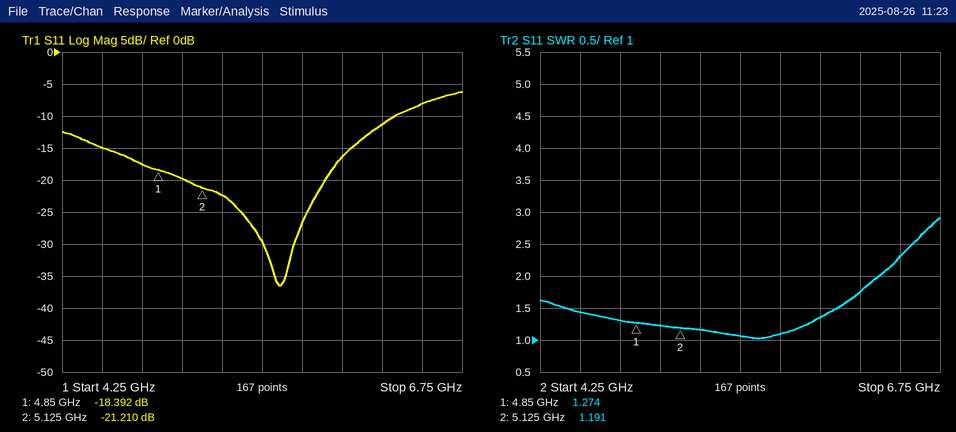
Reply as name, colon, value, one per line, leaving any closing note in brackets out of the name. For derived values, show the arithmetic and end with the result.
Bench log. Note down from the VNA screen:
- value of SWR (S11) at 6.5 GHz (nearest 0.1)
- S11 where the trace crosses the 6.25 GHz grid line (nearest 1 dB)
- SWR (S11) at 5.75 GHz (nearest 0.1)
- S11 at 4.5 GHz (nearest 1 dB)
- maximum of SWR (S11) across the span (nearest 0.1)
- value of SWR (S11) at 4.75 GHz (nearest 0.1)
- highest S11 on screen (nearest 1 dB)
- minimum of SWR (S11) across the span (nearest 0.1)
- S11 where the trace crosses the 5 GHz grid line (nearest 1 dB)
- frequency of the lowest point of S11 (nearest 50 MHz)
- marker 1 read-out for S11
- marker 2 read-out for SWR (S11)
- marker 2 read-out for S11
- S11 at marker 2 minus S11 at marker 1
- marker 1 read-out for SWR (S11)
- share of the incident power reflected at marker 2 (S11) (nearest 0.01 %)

value of SWR (S11) at 6.5 GHz: 2.3
S11 where the trace crosses the 6.25 GHz grid line: -11 dB
SWR (S11) at 5.75 GHz: 1.1
S11 at 4.5 GHz: -15 dB
maximum of SWR (S11) across the span: 2.9
value of SWR (S11) at 4.75 GHz: 1.3
highest S11 on screen: -6 dB
minimum of SWR (S11) across the span: 1.0
S11 where the trace crosses the 5 GHz grid line: -20 dB
frequency of the lowest point of S11: 5.60 GHz
marker 1 read-out for S11: -18.392 dB
marker 2 read-out for SWR: 1.191
marker 2 read-out for S11: -21.210 dB
S11 at marker 2 minus S11 at marker 1: -21.21 − (-18.392) = -2.818 dB
marker 1 read-out for SWR: 1.274
share of the incident power reflected at marker 2 (S11): 10^(-21.21/10) ≈ 0.76 %
